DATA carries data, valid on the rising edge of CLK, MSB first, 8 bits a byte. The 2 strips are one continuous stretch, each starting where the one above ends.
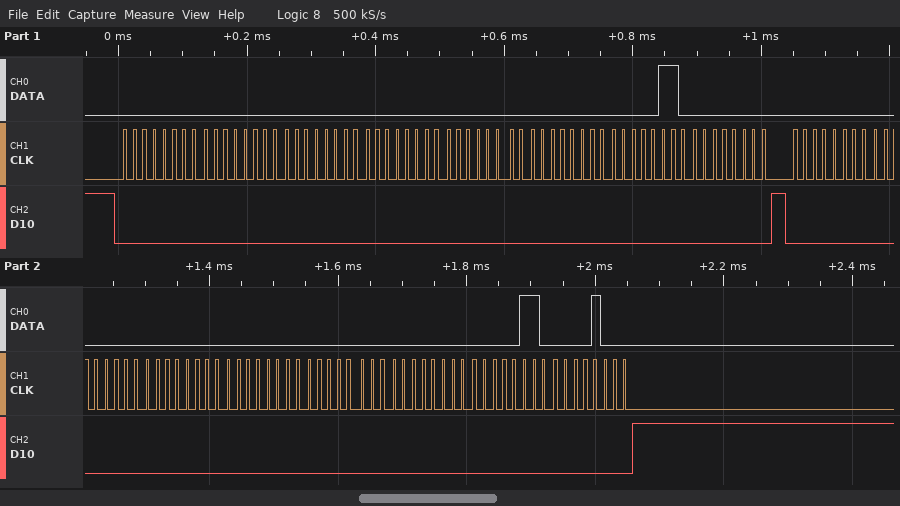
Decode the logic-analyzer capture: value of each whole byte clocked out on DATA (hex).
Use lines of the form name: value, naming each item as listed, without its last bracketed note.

value of each whole byte clocked out on DATA: 00 00 00 00 00 00 06 00 00 00 00 00 00 00 06 08
